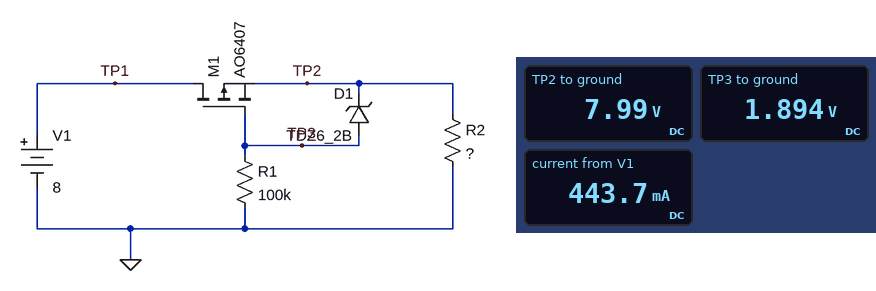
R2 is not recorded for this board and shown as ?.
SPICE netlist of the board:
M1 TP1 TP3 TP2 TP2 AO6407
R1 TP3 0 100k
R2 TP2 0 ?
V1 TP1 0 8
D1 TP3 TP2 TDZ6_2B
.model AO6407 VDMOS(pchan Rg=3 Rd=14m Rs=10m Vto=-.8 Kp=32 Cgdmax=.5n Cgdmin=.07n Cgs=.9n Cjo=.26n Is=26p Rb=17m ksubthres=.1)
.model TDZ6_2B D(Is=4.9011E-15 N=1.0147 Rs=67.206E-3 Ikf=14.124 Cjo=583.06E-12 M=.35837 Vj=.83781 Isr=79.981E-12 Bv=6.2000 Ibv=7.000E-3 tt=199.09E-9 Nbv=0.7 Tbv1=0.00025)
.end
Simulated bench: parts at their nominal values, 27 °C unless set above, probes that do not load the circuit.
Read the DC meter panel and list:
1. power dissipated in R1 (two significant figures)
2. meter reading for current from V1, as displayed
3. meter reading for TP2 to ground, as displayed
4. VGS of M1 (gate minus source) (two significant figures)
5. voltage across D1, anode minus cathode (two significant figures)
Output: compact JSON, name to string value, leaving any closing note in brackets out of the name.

{"power dissipated in R1": "36 µW", "meter reading for current from V1, as displayed": "443.7 mA", "meter reading for TP2 to ground, as displayed": "7.99 V", "VGS of M1 (gate minus source)": "-6.1 V", "voltage across D1, anode minus cathode": "-6.1 V"}
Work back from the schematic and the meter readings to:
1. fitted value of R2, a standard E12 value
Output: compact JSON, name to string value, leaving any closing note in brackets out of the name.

{"fitted value of R2, a standard E12 value": "18 Ω"}
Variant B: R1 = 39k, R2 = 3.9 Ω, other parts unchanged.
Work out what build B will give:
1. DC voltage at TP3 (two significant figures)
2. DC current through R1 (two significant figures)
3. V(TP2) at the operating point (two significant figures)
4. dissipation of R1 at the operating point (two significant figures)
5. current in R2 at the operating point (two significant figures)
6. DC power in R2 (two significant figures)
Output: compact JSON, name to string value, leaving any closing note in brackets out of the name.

{"DC voltage at TP3": "1.8 V", "DC current through R1": "47 µA", "V(TP2) at the operating point": "7.9 V", "dissipation of R1 at the operating point": "86 µW", "current in R2 at the operating point": "2.0 A", "DC power in R2": "16 W"}
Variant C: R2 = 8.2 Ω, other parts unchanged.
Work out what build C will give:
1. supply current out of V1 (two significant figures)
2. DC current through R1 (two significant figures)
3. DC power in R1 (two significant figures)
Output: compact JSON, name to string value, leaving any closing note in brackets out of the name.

{"supply current out of V1": "970 mA", "DC current through R1": "19 µA", "DC power in R1": "35 µW"}
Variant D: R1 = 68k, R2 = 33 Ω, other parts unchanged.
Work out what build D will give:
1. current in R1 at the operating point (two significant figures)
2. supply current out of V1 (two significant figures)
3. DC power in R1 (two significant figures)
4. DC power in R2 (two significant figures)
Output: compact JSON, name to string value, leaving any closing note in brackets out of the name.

{"current in R1 at the operating point": "28 µA", "supply current out of V1": "240 mA", "DC power in R1": "53 µW", "DC power in R2": "1.9 W"}
